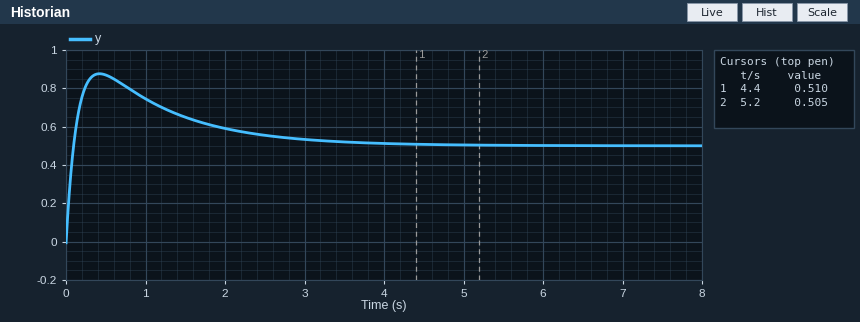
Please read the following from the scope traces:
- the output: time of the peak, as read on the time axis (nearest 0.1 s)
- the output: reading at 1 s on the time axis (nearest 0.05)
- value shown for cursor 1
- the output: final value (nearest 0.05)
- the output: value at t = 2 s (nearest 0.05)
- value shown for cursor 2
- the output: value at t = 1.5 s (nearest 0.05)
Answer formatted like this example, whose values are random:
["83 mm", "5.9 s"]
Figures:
["0.4 s", "0.75", "0.510", "0.50", "0.60", "0.505", "0.65"]
